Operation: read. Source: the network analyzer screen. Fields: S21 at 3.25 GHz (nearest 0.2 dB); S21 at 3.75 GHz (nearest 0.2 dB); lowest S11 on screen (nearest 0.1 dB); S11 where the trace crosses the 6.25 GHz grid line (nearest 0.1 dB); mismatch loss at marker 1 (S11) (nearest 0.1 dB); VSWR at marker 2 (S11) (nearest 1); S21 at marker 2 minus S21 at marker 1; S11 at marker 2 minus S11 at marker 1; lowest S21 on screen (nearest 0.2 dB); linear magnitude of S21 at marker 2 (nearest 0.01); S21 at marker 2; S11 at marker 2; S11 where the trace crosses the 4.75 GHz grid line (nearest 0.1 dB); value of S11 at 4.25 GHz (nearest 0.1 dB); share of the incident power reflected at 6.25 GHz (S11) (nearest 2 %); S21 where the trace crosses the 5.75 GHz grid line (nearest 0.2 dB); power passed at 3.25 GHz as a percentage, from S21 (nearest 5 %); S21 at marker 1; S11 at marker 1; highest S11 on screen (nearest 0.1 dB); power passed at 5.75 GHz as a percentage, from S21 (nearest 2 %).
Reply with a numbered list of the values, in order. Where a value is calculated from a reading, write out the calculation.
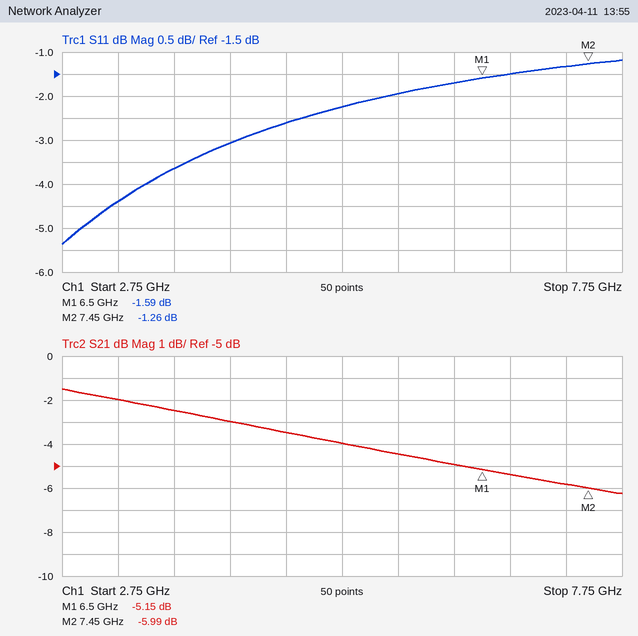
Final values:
1. -2.0 dB
2. -2.4 dB
3. -5.4 dB
4. -1.7 dB
5. −10 log10(1 − 10^(-1.59/10)) ≈ 5.1 dB
6. (1 + 0.8650)/(1 − 0.8650) ≈ 14
7. -5.99 − (-5.15) = -0.84 dB
8. -1.26 − (-1.59) = 0.33 dB
9. -6.2 dB
10. 10^(-5.99/20) ≈ 0.50
11. -5.99 dB
12. -1.26 dB
13. -2.6 dB
14. -3.1 dB
15. 10^(-1.7/10) ≈ 68 %
16. -4.4 dB
17. 10^(-2/10) ≈ 63.1 %, so 65 % to the nearest 5 %
18. -5.15 dB
19. -1.59 dB
20. -1.2 dB
21. 10^(-4.4/10) ≈ 36 %
